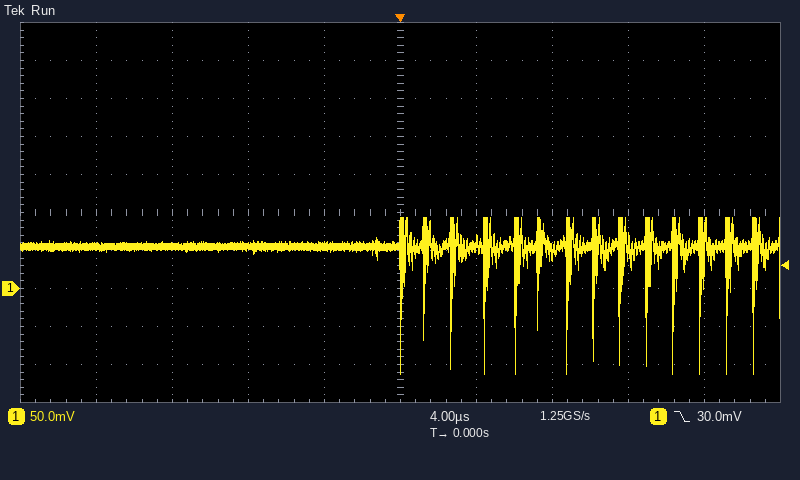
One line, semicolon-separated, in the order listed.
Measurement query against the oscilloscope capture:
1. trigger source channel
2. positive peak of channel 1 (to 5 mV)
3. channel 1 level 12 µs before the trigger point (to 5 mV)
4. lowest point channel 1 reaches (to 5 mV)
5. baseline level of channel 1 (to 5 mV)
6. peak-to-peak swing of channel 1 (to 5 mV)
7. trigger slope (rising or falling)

channel 1; 95 mV; 55 mV; -110 mV; 55 mV; 205 mV; falling
